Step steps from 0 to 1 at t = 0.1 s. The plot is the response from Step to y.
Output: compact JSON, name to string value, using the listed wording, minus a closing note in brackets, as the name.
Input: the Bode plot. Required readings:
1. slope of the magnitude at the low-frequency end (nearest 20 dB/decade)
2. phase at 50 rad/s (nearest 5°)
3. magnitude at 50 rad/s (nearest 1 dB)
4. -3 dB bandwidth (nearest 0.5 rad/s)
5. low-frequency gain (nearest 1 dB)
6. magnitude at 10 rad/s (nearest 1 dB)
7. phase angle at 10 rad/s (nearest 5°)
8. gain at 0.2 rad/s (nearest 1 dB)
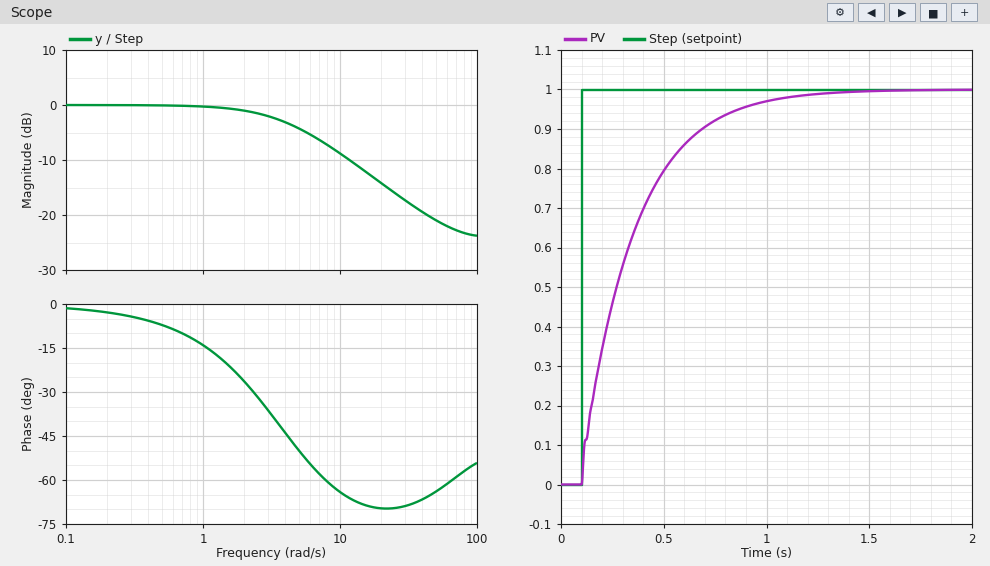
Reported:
{"slope of the magnitude at the low-frequency end": "0 dB/decade", "phase at 50 rad/s": "-65°", "magnitude at 50 rad/s": "-21 dB", "-3 dB bandwidth": "4.0 rad/s", "low-frequency gain": "0 dB", "magnitude at 10 rad/s": "-9 dB", "phase angle at 10 rad/s": "-65°", "gain at 0.2 rad/s": "0 dB"}
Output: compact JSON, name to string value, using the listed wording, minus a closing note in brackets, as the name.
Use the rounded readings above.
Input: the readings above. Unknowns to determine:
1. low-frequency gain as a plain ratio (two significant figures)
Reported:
{"low-frequency gain as a plain ratio": "1.0"}
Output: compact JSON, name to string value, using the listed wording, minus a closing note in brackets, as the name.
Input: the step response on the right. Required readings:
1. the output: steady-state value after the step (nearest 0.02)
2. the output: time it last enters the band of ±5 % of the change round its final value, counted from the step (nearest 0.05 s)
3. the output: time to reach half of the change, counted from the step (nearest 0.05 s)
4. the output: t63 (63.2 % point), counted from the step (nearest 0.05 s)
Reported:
{"the output: steady-state value after the step": "1.00", "the output: time it last enters the band of ±5 % of the change round its final value, counted from the step": "0.75 s", "the output: time to reach half of the change, counted from the step": "0.15 s", "the output: t63 (63.2 % point), counted from the step": "0.25 s"}
